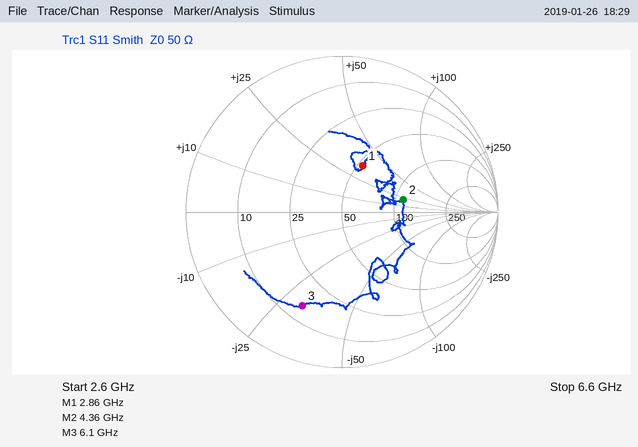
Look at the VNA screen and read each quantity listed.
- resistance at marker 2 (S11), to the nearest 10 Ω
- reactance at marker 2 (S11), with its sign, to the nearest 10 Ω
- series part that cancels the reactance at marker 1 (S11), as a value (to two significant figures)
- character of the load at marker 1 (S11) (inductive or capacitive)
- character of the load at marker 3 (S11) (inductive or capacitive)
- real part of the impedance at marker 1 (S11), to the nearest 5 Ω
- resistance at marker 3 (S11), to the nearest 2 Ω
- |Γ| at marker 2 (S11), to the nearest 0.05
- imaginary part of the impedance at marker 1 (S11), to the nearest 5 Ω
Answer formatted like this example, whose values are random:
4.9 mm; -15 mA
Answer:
110 Ω; +20 Ω; 1.6 pF; inductive; capacitive; 55 Ω; 14 Ω; 0.40; +35 Ω
